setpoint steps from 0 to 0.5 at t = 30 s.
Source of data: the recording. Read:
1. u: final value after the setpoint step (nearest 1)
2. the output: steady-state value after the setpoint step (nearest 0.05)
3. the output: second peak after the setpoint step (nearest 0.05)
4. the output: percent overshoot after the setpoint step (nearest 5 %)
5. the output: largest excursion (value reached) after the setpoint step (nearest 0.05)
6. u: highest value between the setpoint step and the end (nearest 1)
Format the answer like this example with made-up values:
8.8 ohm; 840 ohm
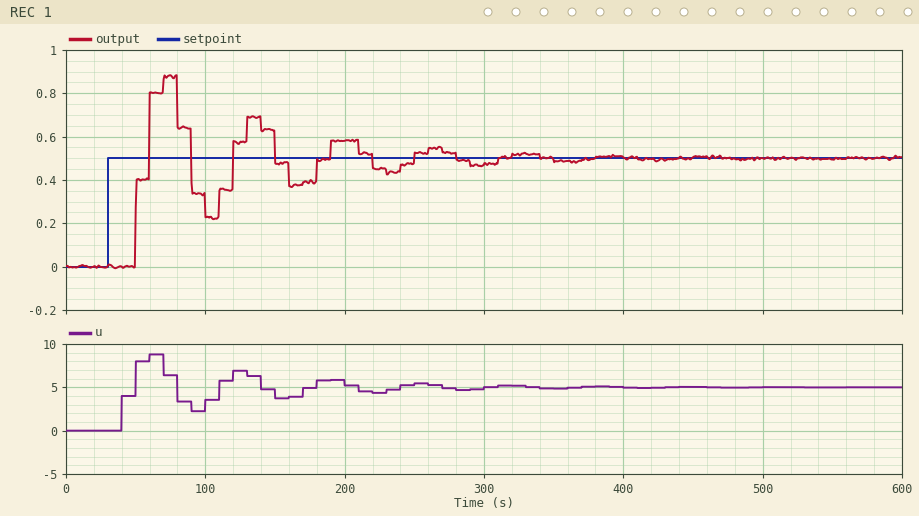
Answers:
5; 0.50; 0.70; 75 %; 0.90; 9
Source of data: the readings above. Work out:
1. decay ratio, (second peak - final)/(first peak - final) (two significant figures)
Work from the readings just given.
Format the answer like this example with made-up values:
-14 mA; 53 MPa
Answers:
0.50
